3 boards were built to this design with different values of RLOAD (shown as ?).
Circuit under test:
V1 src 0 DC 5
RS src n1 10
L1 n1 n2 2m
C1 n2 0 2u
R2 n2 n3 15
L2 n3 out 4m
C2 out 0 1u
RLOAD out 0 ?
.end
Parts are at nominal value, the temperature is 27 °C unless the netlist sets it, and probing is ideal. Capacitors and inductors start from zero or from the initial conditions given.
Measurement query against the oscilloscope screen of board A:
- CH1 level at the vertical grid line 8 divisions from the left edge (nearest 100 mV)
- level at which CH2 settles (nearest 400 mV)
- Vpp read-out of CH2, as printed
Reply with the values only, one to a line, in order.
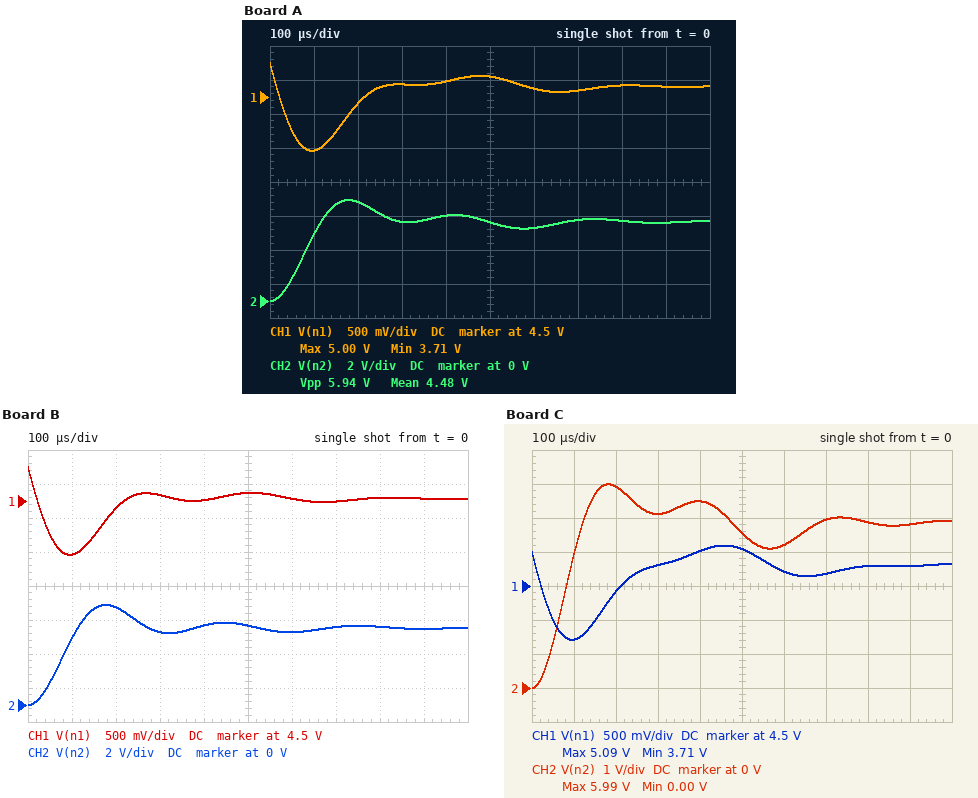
4.7 V
4.8 V
5.94 V
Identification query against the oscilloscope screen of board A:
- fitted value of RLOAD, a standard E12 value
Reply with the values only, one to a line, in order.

120 Ω
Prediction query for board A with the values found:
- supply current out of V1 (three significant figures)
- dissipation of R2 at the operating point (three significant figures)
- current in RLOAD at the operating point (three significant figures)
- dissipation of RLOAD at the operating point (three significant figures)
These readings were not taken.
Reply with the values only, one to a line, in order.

34.5 mA
17.8 mW
34.5 mA
143 mW
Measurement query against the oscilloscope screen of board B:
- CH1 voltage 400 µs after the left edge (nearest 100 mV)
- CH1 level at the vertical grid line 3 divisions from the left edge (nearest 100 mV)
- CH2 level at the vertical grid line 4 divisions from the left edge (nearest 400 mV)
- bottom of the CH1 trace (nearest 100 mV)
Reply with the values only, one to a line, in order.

4.5 V
4.6 V
4.8 V
3.7 V
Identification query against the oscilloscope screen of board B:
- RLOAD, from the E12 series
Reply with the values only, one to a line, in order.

82 Ω
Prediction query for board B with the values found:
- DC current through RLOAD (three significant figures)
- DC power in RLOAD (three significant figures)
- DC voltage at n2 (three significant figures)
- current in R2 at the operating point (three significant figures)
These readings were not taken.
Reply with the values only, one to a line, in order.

46.7 mA
179 mW
4.53 V
46.7 mA
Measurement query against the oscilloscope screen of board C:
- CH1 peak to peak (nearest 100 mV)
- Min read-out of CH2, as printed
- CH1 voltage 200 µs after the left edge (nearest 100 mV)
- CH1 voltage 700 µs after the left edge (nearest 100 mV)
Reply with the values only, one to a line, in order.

1.4 V
0.00 V
4.4 V
4.7 V
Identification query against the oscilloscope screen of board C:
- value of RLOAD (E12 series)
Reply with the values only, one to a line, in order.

220 Ω
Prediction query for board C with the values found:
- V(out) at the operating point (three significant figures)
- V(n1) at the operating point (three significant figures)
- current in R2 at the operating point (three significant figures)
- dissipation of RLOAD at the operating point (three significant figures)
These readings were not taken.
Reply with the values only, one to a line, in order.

4.49 V
4.80 V
20.4 mA
91.6 mW
